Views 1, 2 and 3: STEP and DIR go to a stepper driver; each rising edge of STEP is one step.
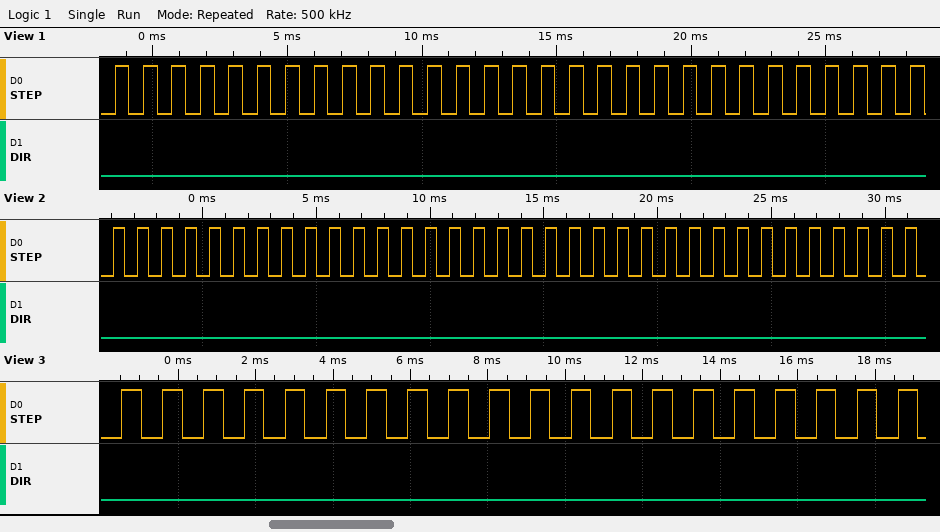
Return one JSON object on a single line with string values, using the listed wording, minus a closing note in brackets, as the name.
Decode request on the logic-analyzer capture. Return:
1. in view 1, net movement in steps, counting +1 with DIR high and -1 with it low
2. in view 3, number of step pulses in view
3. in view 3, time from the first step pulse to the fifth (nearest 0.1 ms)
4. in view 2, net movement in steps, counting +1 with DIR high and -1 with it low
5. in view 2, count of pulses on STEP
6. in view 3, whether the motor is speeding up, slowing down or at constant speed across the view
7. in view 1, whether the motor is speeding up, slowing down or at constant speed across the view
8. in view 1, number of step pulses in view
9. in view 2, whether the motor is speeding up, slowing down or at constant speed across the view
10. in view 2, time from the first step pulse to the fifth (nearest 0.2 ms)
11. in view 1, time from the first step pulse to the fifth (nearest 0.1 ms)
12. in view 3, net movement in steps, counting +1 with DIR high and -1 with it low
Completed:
{"in view 1, net movement in steps, counting +1 with DIR high and -1 with it low": "-29", "in view 3, number of step pulses in view": "20", "in view 3, time from the first step pulse to the fifth": "4.2 ms", "in view 2, net movement in steps, counting +1 with DIR high and -1 with it low": "-34", "in view 2, count of pulses on STEP": "34", "in view 3, whether the motor is speeding up, slowing down or at constant speed across the view": "constant speed", "in view 1, whether the motor is speeding up, slowing down or at constant speed across the view": "constant speed", "in view 1, number of step pulses in view": "29", "in view 2, whether the motor is speeding up, slowing down or at constant speed across the view": "constant speed", "in view 2, time from the first step pulse to the fifth": "4.2 ms", "in view 1, time from the first step pulse to the fifth": "4.2 ms", "in view 3, net movement in steps, counting +1 with DIR high and -1 with it low": "-20"}
